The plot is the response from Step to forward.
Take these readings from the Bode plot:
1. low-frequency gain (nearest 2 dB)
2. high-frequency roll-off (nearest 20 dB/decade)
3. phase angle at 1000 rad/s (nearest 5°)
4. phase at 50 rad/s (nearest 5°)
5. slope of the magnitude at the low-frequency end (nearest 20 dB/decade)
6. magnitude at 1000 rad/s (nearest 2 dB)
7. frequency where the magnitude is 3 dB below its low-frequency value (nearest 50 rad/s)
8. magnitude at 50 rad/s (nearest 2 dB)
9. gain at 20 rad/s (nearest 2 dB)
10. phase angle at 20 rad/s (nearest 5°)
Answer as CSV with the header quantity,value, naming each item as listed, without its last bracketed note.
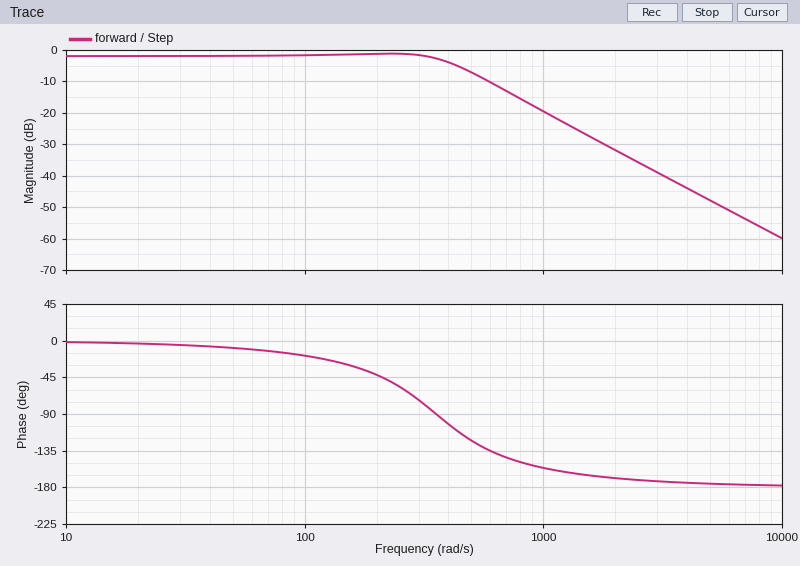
quantity,value
low-frequency gain,-2 dB
high-frequency roll-off,-40 dB/decade
phase angle at 1000 rad/s,-155°
phase at 50 rad/s,-10°
slope of the magnitude at the low-frequency end,0 dB/decade
magnitude at 1000 rad/s,-20 dB
frequency where the magnitude is 3 dB below its low-frequency value,450 rad/s
magnitude at 50 rad/s,-2 dB
gain at 20 rad/s,-2 dB
phase angle at 20 rad/s,-5°
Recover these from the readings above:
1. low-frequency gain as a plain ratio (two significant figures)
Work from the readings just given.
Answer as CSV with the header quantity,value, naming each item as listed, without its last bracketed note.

quantity,value
low-frequency gain as a plain ratio,0.79
